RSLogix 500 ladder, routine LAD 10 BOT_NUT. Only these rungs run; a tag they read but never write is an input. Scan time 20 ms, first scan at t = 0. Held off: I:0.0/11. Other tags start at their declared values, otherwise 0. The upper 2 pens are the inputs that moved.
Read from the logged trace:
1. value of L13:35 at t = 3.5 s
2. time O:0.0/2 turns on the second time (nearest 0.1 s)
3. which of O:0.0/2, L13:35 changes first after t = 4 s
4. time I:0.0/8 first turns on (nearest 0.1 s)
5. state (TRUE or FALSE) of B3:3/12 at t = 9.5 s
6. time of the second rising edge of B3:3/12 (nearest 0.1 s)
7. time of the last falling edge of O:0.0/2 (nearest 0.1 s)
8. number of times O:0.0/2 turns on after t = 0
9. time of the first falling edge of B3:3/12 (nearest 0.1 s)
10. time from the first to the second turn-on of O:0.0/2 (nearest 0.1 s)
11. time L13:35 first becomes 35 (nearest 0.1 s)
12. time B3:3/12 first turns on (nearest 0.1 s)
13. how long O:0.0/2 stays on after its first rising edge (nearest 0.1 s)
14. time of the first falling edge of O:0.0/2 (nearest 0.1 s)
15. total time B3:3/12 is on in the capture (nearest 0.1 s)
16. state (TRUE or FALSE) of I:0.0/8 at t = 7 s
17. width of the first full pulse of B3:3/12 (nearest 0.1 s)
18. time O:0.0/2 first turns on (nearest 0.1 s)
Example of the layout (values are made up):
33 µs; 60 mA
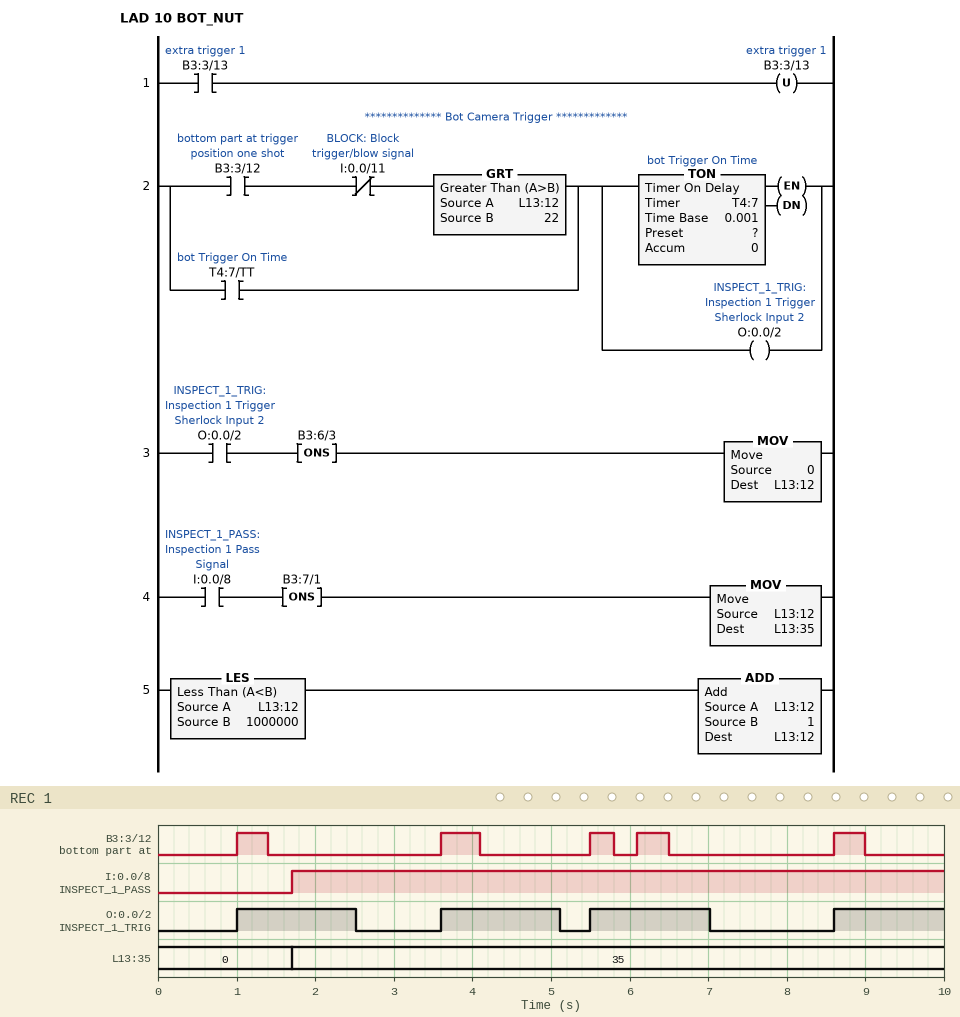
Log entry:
35; 3.6 s; O:0.0/2; 1.7 s; FALSE; 3.6 s; 7.0 s; 4; 1.4 s; 2.6 s; 1.7 s; 1.0 s; 1.5 s; 2.5 s; 2.0 s; TRUE; 0.4 s; 1.0 s
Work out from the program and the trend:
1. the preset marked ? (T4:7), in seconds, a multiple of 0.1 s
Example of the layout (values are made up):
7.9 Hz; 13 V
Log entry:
1.5 s
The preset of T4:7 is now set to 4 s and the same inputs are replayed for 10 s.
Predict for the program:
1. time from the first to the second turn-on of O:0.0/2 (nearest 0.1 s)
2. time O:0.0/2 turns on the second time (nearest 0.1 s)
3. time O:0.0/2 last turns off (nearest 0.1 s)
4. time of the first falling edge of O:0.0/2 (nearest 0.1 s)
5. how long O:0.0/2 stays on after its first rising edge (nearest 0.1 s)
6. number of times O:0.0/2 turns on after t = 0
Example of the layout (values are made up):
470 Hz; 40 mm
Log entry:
4.5 s; 5.5 s; 9.5 s; 5.0 s; 4.0 s; 2
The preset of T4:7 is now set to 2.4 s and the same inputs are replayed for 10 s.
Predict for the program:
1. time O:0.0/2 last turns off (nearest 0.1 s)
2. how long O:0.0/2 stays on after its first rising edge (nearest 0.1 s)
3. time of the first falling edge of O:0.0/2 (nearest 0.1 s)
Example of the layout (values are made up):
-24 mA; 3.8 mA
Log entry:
8.5 s; 2.4 s; 3.4 s
